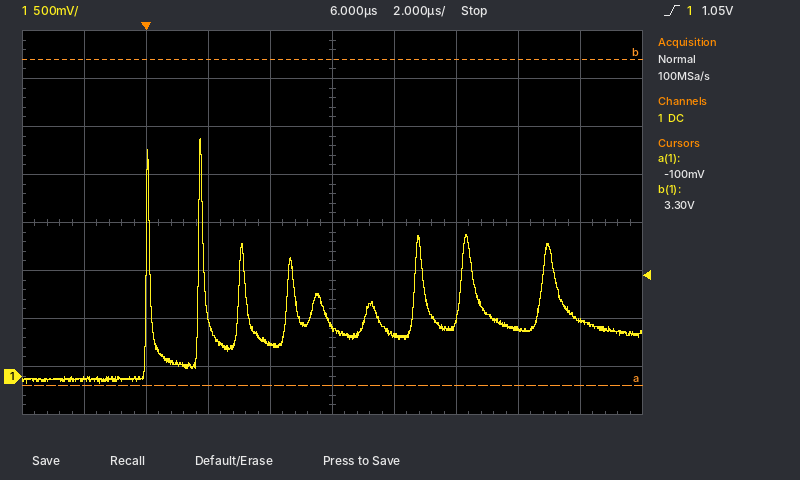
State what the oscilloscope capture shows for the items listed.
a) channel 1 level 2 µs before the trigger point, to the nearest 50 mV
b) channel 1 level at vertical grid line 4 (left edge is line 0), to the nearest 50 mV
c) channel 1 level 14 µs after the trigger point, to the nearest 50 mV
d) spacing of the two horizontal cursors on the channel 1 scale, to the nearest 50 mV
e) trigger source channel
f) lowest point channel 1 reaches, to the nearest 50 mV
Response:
-50 mV
350 mV
600 mV
3.40 V
channel 1
-100 mV
